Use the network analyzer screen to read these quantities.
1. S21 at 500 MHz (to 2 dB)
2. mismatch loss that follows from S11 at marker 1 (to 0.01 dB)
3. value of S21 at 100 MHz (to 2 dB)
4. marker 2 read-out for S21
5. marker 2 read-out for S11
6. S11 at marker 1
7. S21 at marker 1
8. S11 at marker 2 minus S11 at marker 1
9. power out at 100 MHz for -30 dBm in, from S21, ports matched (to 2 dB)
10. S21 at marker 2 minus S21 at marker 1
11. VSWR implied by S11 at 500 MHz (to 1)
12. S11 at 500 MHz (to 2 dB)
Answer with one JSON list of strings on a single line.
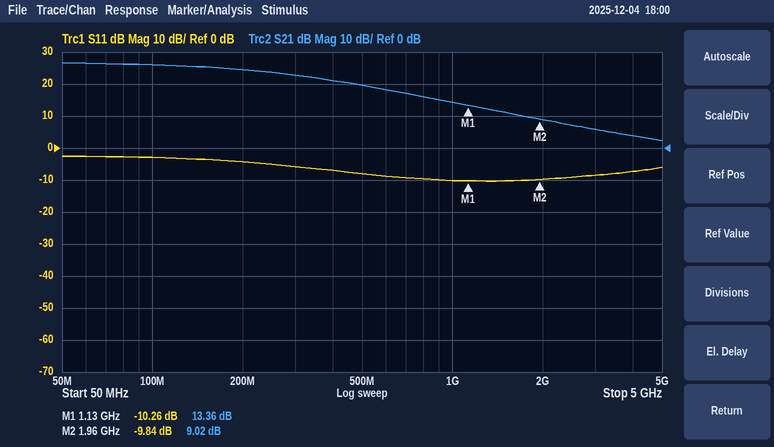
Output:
["20 dB", "0.43 dB", "26 dB", "9.02 dB", "-9.84 dB", "-10.26 dB", "13.36 dB", "0.42 dB", "-4 dBm", "-4.34 dB", "2", "-8 dB"]
